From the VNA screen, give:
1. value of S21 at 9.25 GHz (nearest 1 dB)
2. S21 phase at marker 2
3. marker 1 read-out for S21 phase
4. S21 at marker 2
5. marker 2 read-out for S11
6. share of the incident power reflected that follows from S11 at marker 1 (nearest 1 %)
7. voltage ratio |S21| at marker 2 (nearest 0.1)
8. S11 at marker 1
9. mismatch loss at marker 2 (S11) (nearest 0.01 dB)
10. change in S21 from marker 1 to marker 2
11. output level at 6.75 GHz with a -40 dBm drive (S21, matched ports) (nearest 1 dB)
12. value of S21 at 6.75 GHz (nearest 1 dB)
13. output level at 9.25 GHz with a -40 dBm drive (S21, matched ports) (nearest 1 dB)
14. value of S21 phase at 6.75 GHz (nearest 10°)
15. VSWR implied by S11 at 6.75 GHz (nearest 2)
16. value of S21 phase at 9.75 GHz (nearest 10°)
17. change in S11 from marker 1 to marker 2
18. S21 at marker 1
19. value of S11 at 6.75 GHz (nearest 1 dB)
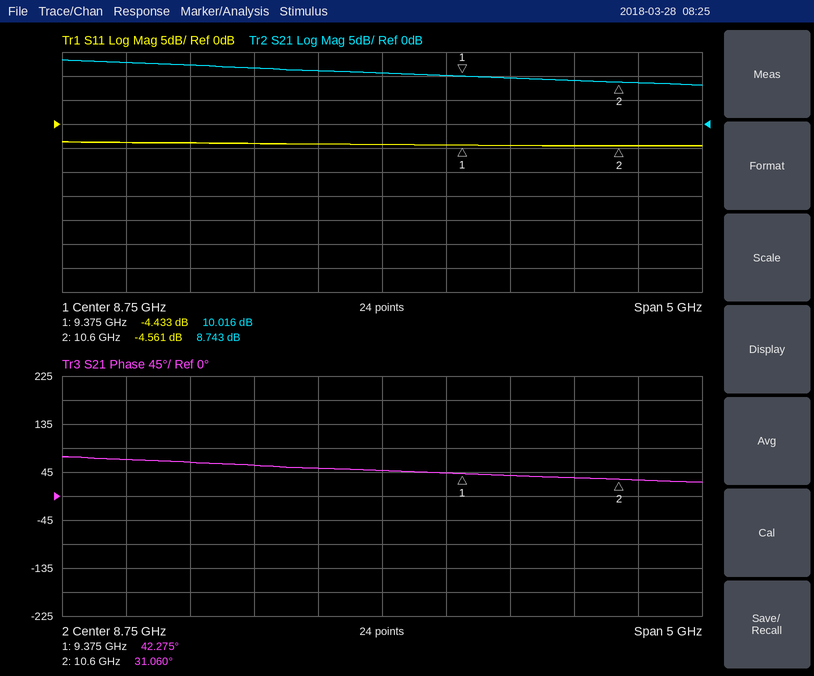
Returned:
10 dB
31.060°
42.275°
8.743 dB
-4.561 dB
36 %
2.7
-4.433 dB
1.87 dB
-1.273 dB
-27 dBm
13 dB
-30 dBm
70°
4
40°
-0.128 dB
10.016 dB
-4 dB
